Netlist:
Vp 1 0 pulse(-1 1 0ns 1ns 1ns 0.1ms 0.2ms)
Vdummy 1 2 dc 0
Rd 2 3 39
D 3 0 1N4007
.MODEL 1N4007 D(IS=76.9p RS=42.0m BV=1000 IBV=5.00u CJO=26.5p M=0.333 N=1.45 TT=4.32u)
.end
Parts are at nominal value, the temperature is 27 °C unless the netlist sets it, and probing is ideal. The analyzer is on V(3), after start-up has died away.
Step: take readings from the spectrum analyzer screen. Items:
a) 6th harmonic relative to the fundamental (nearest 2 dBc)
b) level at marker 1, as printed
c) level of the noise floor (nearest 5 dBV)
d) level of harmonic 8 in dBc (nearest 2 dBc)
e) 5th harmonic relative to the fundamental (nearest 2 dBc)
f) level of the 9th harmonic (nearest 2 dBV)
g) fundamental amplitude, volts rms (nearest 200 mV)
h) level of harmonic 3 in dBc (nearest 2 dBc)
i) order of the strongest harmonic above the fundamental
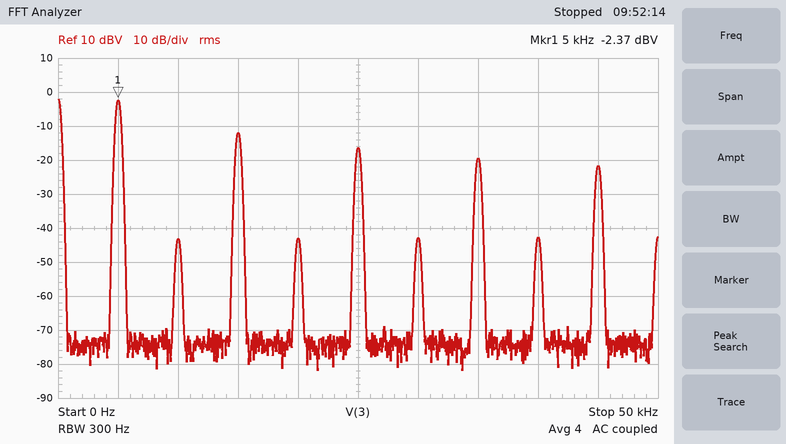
-40 dBc
-2.37 dBV
-75 dBV
-40 dBc
-14 dBc
-22 dBV
800 mV
-10 dBc
3
